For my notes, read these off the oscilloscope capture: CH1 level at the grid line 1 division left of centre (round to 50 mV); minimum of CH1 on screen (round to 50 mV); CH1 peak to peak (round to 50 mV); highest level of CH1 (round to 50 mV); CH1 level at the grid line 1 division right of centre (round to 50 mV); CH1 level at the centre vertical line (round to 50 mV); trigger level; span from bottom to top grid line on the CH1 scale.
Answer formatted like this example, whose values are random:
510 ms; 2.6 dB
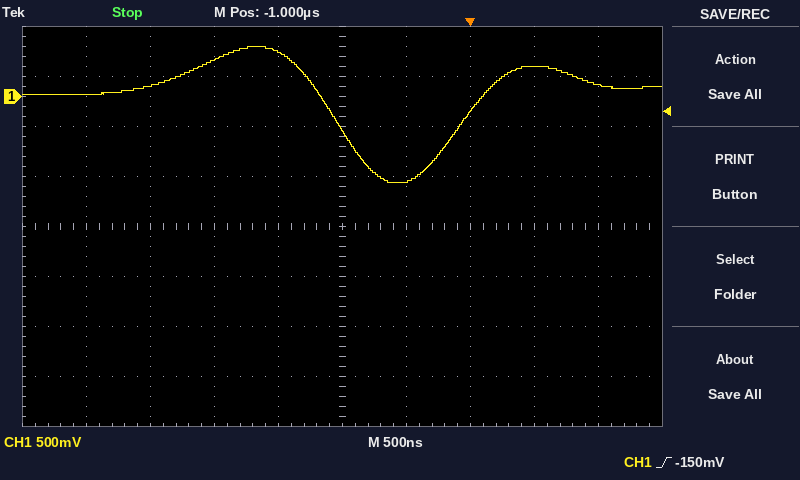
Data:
450 mV; -850 mV; 1.35 V; 500 mV; -850 mV; -350 mV; -150 mV; 4 V
